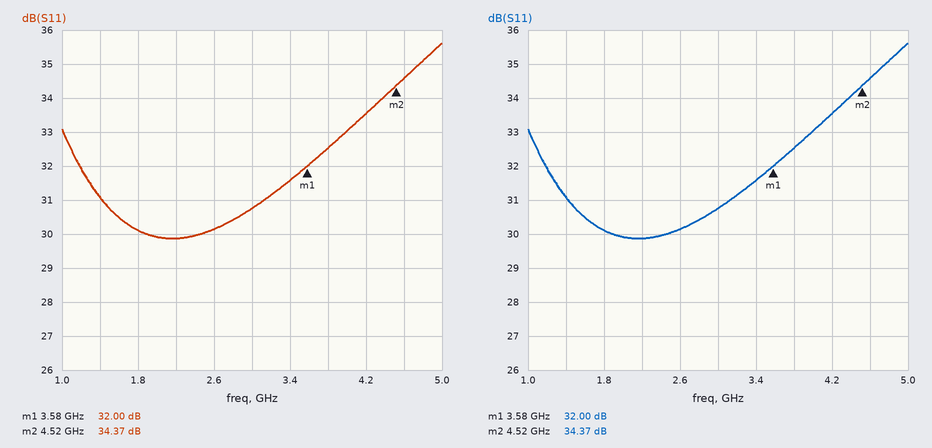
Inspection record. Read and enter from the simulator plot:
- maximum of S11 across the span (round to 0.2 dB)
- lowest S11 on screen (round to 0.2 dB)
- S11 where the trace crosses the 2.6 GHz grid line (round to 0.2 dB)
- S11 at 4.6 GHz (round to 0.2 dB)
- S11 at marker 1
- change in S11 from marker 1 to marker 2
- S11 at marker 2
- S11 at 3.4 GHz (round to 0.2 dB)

35.6 dB
29.8 dB
30.2 dB
34.6 dB
32.00 dB
2.37 dB
34.37 dB
31.6 dB
